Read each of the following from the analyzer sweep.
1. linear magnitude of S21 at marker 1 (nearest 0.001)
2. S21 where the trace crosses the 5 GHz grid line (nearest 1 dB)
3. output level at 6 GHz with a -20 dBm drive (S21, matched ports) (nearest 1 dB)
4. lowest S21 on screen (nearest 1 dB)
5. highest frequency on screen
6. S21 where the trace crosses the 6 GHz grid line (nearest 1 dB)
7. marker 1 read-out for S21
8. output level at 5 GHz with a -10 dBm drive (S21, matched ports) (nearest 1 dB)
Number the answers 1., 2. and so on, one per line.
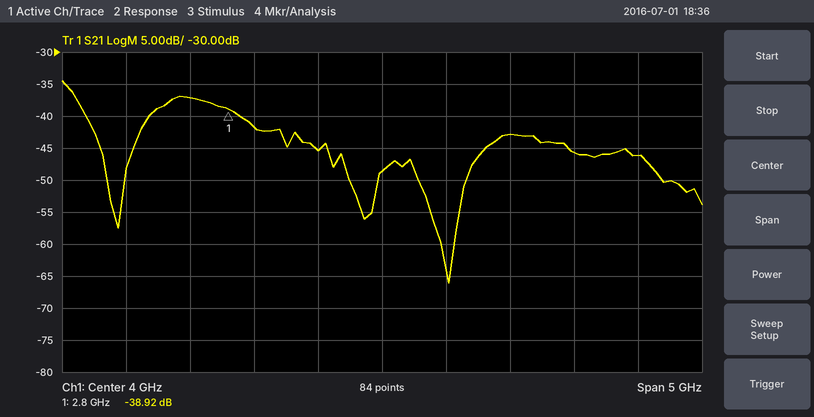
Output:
1. 0.011
2. -43 dB
3. -66 dBm
4. -66 dB
5. 6.5 GHz
6. -46 dB
7. -38.92 dB
8. -53 dBm
